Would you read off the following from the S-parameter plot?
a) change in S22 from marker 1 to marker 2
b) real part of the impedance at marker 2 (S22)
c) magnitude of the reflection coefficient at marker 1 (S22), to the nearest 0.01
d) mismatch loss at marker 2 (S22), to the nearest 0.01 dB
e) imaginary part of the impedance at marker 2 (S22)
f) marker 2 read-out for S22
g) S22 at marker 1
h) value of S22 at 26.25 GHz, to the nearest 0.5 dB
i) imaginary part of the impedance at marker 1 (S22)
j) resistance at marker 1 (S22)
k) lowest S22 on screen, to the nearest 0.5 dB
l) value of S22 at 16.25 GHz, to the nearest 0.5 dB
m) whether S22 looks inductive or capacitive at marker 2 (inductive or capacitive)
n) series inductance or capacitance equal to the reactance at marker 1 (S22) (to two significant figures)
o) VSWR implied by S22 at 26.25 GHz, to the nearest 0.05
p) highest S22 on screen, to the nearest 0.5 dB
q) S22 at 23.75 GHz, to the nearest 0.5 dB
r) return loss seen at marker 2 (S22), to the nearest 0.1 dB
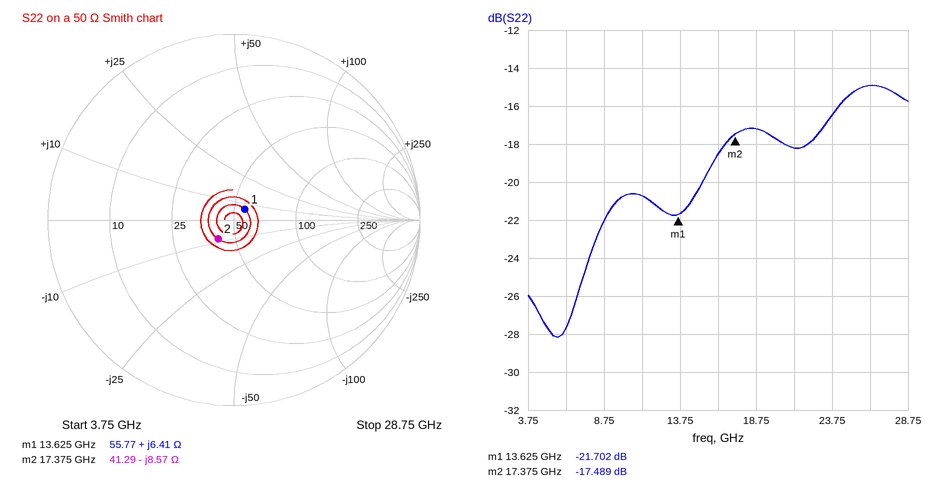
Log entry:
4.213 dB
41.29 Ω
0.08
0.08 dB
-8.57 Ω
-17.489 dB
-21.702 dB
-15.0 dB
+6.41 Ω
55.77 Ω
-28.0 dB
-18.5 dB
capacitive
75 pH
1.45
-15.0 dB
-16.5 dB
17.5 dB
